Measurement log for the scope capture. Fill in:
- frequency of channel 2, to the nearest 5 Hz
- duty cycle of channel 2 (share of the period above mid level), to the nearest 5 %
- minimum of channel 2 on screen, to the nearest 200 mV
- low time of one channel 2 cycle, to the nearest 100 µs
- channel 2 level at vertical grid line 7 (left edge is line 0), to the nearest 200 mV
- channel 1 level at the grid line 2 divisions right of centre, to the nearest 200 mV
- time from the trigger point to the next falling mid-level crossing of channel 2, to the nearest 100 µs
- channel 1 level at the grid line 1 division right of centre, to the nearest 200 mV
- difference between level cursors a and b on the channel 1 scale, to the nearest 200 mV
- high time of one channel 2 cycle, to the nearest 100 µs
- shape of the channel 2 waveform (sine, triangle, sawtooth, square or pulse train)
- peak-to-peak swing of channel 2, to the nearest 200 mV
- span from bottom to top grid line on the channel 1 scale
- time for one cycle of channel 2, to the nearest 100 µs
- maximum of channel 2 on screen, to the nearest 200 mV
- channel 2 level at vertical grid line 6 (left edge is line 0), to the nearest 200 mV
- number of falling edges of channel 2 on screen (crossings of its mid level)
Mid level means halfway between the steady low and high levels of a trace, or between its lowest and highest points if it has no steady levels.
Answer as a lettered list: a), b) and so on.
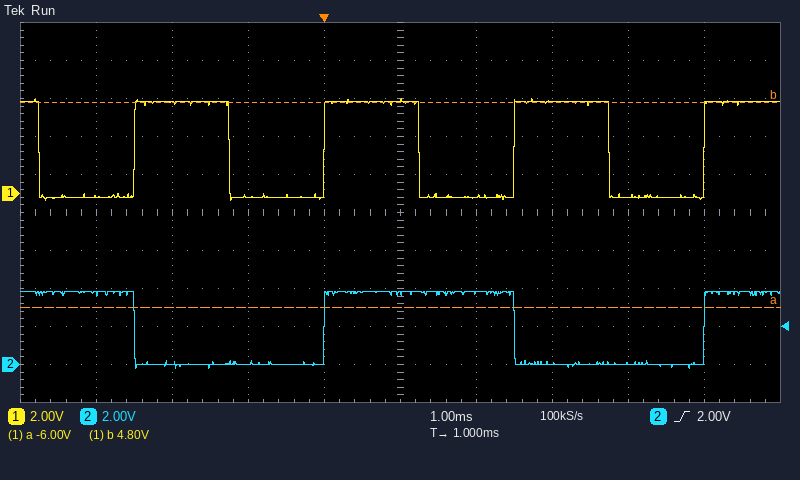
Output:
a) 200 Hz
b) 50 %
c) -200 mV
d) 2.5 ms
e) 0.0 V
f) 4.8 V
g) 2.5 ms
h) -200 mV
i) 10.8 V
j) 2.5 ms
k) square
l) 4.0 V
m) 20 V
n) 5.0 ms
o) 3.8 V
p) 3.8 V
q) 2
